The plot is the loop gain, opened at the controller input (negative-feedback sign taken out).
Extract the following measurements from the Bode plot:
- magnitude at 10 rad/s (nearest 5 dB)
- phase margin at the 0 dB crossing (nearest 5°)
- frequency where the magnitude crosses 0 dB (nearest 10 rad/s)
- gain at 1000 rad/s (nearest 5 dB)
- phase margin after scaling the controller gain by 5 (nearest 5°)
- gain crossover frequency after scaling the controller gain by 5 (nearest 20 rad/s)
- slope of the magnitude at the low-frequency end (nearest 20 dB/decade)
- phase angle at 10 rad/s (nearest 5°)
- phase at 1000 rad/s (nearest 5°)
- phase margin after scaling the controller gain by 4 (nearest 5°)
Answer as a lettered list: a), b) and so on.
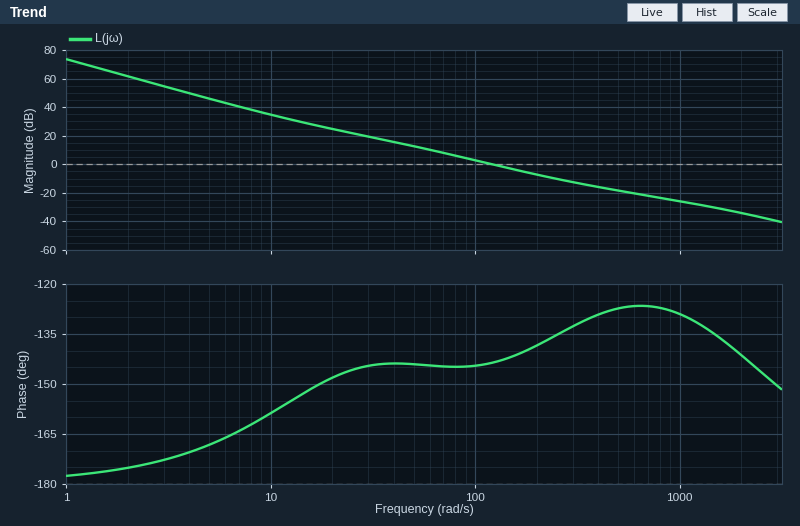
a) 35 dB
b) 35°
c) 120 rad/s
d) -25 dB
e) 50°
f) 340 rad/s
g) -40 dB/decade
h) -160°
i) -130°
j) 45°
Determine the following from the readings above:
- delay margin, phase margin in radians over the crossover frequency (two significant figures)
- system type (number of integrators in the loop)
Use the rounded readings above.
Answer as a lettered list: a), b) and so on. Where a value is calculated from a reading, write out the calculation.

a) 35 × π / 180 / 120 = 0.0051 s
b) 2
